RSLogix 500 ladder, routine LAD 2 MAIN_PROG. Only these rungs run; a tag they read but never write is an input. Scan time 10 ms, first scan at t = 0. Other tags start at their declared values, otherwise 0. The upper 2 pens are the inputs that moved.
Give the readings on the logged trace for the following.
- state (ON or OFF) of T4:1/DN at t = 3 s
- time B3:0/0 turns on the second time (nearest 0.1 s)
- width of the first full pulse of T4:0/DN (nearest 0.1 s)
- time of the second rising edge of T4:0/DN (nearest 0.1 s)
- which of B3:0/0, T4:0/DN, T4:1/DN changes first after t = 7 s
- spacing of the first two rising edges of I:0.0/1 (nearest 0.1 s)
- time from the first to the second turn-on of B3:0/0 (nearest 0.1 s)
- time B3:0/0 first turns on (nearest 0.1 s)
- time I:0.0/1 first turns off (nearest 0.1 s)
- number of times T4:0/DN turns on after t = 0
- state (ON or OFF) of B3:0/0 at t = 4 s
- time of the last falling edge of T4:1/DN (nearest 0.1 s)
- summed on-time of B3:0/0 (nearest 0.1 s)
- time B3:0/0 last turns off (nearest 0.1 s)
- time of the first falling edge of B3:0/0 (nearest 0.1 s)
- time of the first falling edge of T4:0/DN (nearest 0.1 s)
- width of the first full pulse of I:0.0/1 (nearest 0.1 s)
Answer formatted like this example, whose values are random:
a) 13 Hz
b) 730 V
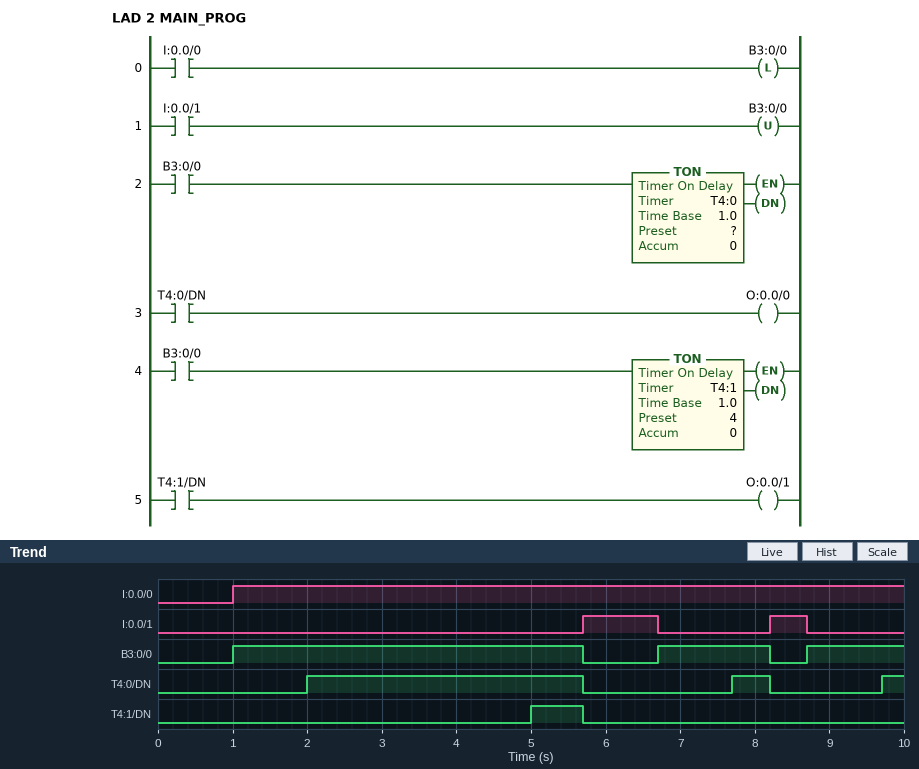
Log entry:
a) OFF
b) 6.7 s
c) 3.7 s
d) 7.7 s
e) T4:0/DN
f) 2.5 s
g) 5.7 s
h) 1.0 s
i) 6.7 s
j) 3
k) ON
l) 5.7 s
m) 7.5 s
n) 8.2 s
o) 5.7 s
p) 5.7 s
q) 1.0 s
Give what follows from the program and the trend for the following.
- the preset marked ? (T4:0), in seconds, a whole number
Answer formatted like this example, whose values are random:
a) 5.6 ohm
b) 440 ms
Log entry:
a) 1 s
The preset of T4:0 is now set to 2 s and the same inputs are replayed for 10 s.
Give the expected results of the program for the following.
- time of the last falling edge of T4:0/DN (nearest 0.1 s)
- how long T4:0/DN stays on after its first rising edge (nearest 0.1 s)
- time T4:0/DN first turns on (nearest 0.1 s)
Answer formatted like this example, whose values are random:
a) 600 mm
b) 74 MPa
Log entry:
a) 5.7 s
b) 2.7 s
c) 3.0 s
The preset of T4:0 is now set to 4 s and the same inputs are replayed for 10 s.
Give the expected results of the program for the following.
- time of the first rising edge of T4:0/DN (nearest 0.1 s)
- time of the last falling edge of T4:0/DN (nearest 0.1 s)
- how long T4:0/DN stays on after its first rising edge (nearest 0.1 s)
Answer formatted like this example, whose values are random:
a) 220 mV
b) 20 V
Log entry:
a) 5.0 s
b) 5.7 s
c) 0.7 s
